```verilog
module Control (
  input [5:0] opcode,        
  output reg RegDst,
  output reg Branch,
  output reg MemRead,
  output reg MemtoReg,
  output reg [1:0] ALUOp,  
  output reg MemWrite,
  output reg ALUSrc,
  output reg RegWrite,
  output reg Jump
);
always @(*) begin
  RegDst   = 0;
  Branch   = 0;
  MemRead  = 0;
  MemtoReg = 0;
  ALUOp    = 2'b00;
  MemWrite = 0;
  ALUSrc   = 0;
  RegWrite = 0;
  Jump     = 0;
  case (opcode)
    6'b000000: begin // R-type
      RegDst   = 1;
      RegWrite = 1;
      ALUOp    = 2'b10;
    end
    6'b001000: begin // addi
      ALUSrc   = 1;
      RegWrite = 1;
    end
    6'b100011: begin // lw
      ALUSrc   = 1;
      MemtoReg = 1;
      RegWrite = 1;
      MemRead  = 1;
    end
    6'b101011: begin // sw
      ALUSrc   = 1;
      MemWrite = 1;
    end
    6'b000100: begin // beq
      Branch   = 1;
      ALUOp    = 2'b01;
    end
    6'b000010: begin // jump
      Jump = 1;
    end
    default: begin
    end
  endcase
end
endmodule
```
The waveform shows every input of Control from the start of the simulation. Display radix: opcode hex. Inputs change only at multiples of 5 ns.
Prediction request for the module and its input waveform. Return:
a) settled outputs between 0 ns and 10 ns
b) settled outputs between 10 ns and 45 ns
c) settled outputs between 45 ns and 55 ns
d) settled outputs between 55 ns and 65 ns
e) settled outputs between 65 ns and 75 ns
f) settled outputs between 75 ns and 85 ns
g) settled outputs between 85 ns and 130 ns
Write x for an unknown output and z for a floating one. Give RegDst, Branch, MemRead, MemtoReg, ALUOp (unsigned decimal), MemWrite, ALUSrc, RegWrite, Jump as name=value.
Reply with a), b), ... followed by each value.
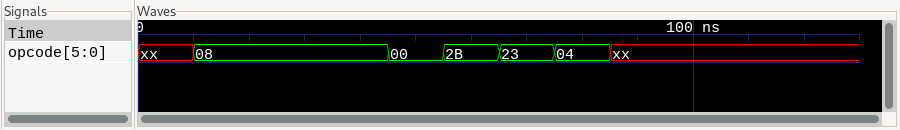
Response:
a) RegDst=x, Branch=x, MemRead=x, MemtoReg=x, ALUOp=x, MemWrite=x, ALUSrc=x, RegWrite=x, Jump=x
b) RegDst=0, Branch=0, MemRead=0, MemtoReg=0, ALUOp=0, MemWrite=0, ALUSrc=1, RegWrite=1, Jump=0
c) RegDst=1, Branch=0, MemRead=0, MemtoReg=0, ALUOp=2, MemWrite=0, ALUSrc=0, RegWrite=1, Jump=0
d) RegDst=0, Branch=0, MemRead=0, MemtoReg=0, ALUOp=0, MemWrite=1, ALUSrc=1, RegWrite=0, Jump=0
e) RegDst=0, Branch=0, MemRead=1, MemtoReg=1, ALUOp=0, MemWrite=0, ALUSrc=1, RegWrite=1, Jump=0
f) RegDst=0, Branch=1, MemRead=0, MemtoReg=0, ALUOp=1, MemWrite=0, ALUSrc=0, RegWrite=0, Jump=0
g) RegDst=0, Branch=0, MemRead=0, MemtoReg=0, ALUOp=0, MemWrite=0, ALUSrc=0, RegWrite=0, Jump=0
